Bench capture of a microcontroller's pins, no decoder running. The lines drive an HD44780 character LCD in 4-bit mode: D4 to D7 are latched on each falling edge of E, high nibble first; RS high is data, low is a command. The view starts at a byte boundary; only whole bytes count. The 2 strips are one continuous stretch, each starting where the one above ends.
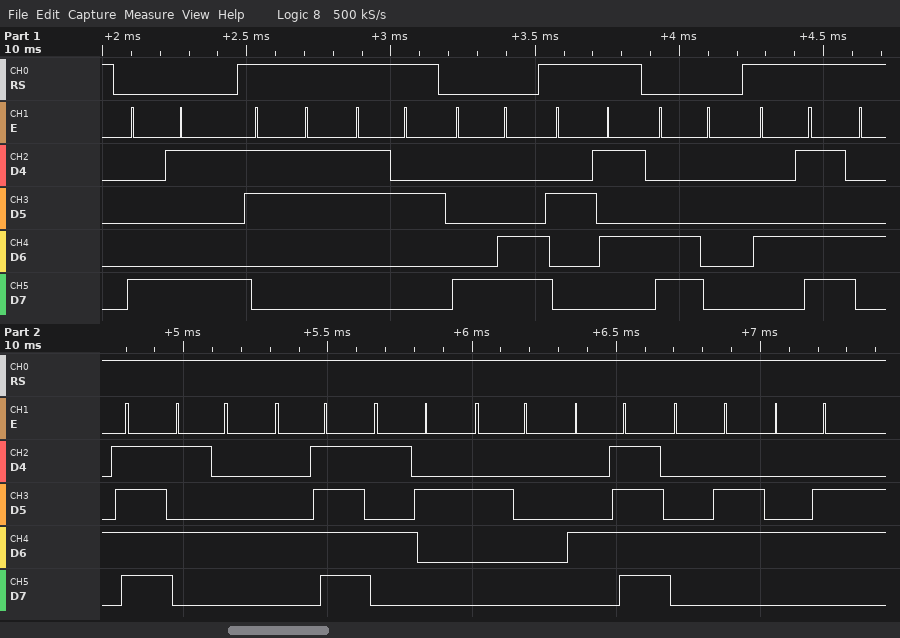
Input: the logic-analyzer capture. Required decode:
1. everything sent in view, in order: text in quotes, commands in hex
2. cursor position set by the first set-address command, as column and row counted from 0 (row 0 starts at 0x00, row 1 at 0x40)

0x89 "32" 0x8C "%" 0xC0 "MOTOR OFF"
column 9, row 0
